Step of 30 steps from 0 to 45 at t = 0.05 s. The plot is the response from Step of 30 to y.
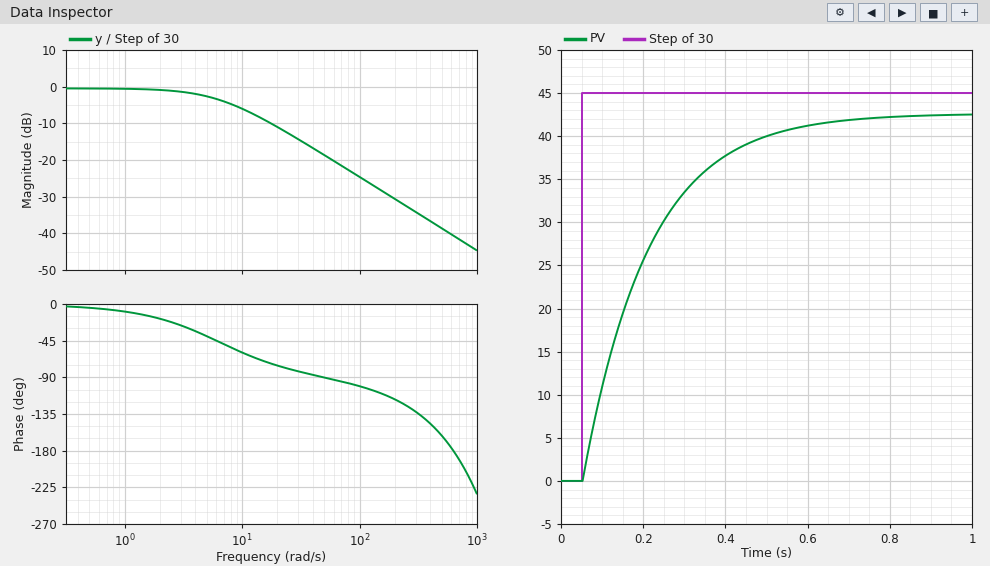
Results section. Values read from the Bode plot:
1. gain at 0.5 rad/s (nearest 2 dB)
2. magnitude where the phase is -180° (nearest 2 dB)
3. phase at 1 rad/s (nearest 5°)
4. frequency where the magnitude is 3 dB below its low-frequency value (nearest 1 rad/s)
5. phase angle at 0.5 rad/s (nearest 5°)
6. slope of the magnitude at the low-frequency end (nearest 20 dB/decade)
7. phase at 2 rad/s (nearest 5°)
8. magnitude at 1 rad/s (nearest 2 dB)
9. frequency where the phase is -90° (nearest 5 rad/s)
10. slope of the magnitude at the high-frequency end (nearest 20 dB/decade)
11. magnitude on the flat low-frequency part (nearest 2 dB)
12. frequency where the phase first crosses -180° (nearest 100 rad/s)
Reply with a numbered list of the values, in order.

1. 0 dB
2. -40 dB
3. -10°
4. 6 rad/s
5. -5°
6. 0 dB/decade
7. -20°
8. 0 dB
9. 50 rad/s
10. -20 dB/decade
11. 0 dB
12. 600 rad/s
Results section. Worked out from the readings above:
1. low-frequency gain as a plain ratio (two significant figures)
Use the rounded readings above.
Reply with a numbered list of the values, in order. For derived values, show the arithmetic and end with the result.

1. 10^(0 / 20) = 1.0
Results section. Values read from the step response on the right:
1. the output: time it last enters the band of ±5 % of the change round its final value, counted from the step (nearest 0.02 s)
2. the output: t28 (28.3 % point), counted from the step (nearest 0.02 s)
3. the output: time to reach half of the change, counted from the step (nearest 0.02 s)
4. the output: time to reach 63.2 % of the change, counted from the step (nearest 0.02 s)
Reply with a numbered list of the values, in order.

1. 0.48 s
2. 0.06 s
3. 0.12 s
4. 0.16 s
